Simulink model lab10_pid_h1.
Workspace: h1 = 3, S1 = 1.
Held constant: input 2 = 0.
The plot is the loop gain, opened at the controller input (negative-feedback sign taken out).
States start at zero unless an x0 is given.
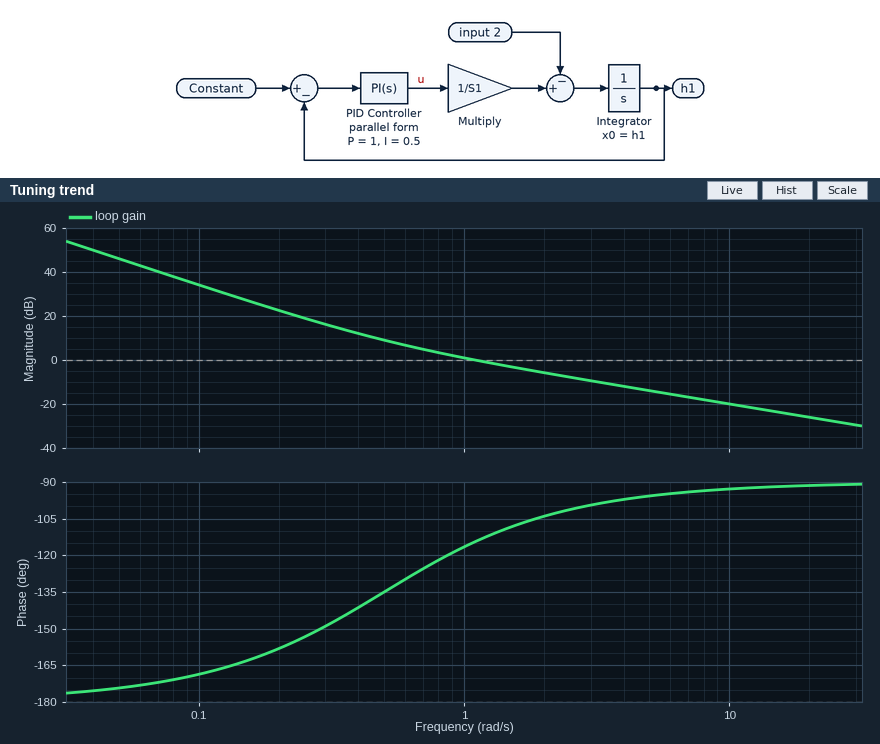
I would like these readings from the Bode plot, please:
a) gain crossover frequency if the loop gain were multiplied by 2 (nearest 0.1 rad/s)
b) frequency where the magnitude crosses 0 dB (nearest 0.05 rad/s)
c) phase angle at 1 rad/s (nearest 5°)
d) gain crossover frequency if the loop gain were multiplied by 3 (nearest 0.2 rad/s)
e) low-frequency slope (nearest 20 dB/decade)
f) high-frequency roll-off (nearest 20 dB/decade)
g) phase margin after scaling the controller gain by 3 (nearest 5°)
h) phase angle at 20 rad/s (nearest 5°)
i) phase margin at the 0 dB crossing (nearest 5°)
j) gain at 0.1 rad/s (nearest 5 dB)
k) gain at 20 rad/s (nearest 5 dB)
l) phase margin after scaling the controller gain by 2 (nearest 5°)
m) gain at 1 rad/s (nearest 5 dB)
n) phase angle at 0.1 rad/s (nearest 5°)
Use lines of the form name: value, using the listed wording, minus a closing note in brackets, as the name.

gain crossover frequency if the loop gain were multiplied by 2: 2.1 rad/s
frequency where the magnitude crosses 0 dB: 1.10 rad/s
phase angle at 1 rad/s: -115°
gain crossover frequency if the loop gain were multiplied by 3: 3.0 rad/s
low-frequency slope: -40 dB/decade
high-frequency roll-off: -20 dB/decade
phase margin after scaling the controller gain by 3: 80°
phase angle at 20 rad/s: -90°
phase margin at the 0 dB crossing: 65°
gain at 0.1 rad/s: 35 dB
gain at 20 rad/s: -25 dB
phase margin after scaling the controller gain by 2: 75°
gain at 1 rad/s: 0 dB
phase angle at 0.1 rad/s: -170°
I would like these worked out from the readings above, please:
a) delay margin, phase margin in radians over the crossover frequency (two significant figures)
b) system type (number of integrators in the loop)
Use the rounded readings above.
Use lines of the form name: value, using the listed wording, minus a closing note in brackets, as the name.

delay margin, phase margin in radians over the crossover frequency: 1.0 s
system type: 2
